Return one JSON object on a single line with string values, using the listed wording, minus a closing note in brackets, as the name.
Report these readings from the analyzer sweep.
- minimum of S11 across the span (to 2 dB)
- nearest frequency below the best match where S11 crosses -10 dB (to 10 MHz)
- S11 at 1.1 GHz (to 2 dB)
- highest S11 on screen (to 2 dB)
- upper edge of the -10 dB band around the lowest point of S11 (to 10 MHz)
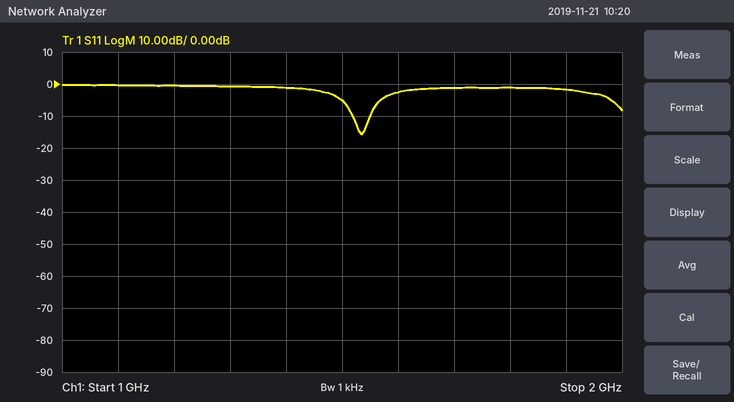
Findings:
{"minimum of S11 across the span": "-16 dB", "nearest frequency below the best match where S11 crosses -10 dB": "1.52 GHz", "S11 at 1.1 GHz": "0 dB", "highest S11 on screen": "0 dB", "upper edge of the -10 dB band around the lowest point of S11": "1.55 GHz"}
